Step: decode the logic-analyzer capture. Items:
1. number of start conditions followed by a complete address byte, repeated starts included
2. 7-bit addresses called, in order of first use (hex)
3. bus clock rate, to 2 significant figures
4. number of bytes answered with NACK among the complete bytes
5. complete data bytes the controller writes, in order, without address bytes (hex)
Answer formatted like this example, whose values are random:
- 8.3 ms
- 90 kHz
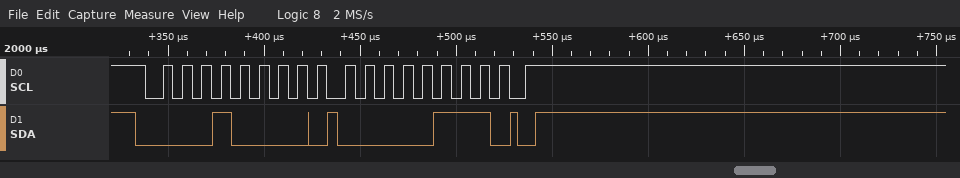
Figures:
- 1
- 0x08
- 100 kHz
- 0
- 07
